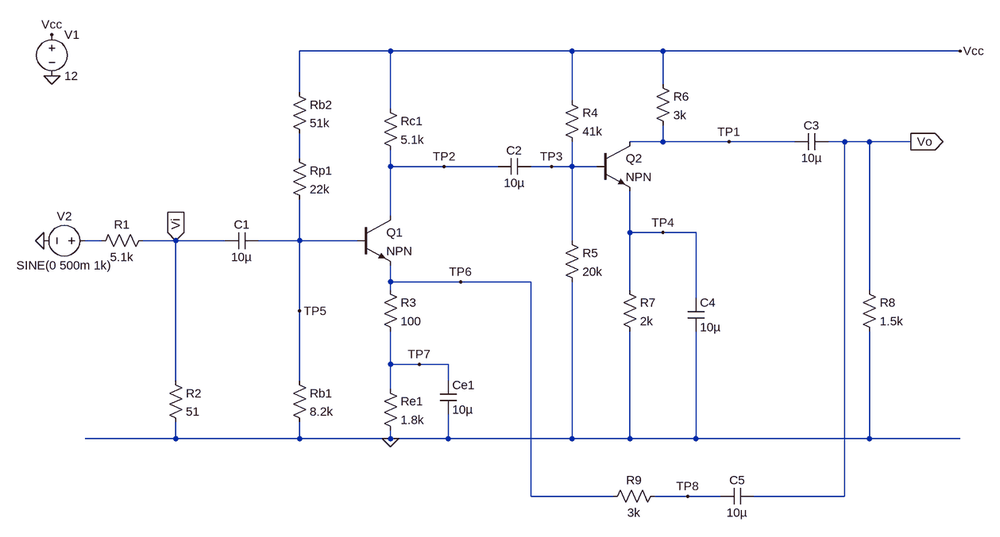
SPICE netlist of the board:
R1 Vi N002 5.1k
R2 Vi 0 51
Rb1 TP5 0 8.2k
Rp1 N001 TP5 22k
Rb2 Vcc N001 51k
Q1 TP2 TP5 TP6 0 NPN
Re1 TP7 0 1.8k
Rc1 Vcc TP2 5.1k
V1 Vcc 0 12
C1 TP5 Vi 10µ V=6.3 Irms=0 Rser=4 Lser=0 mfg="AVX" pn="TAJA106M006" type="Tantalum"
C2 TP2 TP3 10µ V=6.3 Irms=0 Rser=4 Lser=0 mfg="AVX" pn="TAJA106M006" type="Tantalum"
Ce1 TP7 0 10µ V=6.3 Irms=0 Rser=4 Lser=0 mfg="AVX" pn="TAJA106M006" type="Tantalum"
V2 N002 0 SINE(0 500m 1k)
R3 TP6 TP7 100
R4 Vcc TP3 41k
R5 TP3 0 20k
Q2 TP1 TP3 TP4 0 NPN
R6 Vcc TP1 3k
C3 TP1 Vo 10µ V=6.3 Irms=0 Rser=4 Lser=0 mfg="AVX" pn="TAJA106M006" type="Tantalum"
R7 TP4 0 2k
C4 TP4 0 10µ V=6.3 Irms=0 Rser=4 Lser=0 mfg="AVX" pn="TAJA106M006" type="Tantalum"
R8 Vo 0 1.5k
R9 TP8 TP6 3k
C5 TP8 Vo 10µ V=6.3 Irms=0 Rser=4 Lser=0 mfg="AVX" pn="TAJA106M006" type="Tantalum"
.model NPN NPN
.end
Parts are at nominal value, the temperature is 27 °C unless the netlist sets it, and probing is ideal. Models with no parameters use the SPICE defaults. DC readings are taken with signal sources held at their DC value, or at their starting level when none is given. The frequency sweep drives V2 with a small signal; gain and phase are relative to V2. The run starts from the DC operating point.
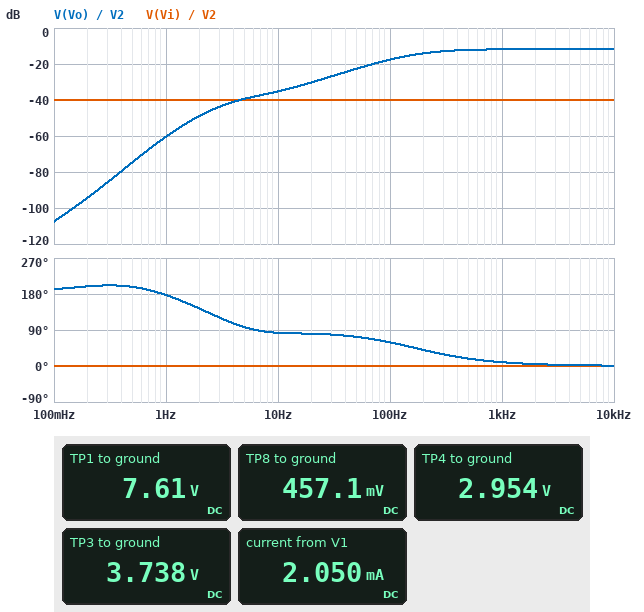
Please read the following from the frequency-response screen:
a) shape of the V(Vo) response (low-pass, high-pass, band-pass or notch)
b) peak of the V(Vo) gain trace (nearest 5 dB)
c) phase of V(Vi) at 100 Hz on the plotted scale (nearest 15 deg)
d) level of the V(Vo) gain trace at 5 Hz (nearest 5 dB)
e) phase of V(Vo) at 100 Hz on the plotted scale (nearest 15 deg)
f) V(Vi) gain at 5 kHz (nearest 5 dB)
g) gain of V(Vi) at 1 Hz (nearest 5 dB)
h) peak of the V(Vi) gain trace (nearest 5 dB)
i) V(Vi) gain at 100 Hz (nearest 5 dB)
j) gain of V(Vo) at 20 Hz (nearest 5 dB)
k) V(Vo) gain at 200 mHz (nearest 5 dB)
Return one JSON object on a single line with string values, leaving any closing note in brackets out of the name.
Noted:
{"shape of the V(Vo) response": "high-pass", "peak of the V(Vo) gain trace": "-10 dB", "phase of V(Vi) at 100 Hz on the plotted scale": "0 deg", "level of the V(Vo) gain trace at 5 Hz": "-40 dB", "phase of V(Vo) at 100 Hz on the plotted scale": "60 deg", "V(Vi) gain at 5 kHz": "-40 dB", "gain of V(Vi) at 1 Hz": "-40 dB", "peak of the V(Vi) gain trace": "-40 dB", "V(Vi) gain at 100 Hz": "-40 dB", "gain of V(Vo) at 20 Hz": "-30 dB", "V(Vo) gain at 200 mHz": "-95 dB"}
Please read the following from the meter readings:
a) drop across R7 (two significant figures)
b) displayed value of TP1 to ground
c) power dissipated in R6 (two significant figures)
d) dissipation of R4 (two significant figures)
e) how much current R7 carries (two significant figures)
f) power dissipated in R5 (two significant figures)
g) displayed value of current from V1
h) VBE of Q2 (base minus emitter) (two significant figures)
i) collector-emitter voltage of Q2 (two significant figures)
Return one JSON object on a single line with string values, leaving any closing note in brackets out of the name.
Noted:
{"drop across R7": "3.0 V", "displayed value of TP1 to ground": "7.61 V", "power dissipated in R6": "6.4 mW", "dissipation of R4": "1.7 mW", "how much current R7 carries": "1.5 mA", "power dissipated in R5": "700 µW", "displayed value of current from V1": "2.050 mA", "VBE of Q2 (base minus emitter)": "780 mV", "collector-emitter voltage of Q2": "4.7 V"}
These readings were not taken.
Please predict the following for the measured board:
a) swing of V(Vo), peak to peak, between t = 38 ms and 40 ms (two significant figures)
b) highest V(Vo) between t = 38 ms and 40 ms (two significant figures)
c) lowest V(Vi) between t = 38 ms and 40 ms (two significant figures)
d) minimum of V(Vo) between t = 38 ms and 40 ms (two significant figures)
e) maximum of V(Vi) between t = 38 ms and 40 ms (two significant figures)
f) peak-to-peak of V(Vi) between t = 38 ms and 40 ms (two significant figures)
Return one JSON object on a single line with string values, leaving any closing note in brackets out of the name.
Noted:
{"swing of V(Vo), peak to peak, between t = 38 ms and 40 ms": "260 mV", "highest V(Vo) between t = 38 ms and 40 ms": "130 mV", "lowest V(Vi) between t = 38 ms and 40 ms": "-4.9 mV", "minimum of V(Vo) between t = 38 ms and 40 ms": "-130 mV", "maximum of V(Vi) between t = 38 ms and 40 ms": "4.9 mV", "peak-to-peak of V(Vi) between t = 38 ms and 40 ms": "9.8 mV"}
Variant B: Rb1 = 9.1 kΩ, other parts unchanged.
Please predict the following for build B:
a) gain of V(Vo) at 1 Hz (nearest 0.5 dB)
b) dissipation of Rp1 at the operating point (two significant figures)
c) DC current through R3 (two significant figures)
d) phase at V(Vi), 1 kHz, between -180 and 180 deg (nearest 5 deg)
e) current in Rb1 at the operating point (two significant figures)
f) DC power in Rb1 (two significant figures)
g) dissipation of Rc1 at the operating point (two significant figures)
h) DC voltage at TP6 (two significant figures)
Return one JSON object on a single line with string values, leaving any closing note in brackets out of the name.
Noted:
{"gain of V(Vo) at 1 Hz": "-59.5 dB", "dissipation of Rp1 at the operating point": "470 µW", "DC current through R3": "300 µA", "phase at V(Vi), 1 kHz, between -180 and 180 deg": "0 deg", "current in Rb1 at the operating point": "140 µA", "DC power in Rb1": "190 µW", "dissipation of Rc1 at the operating point": "440 µW", "DC voltage at TP6": "560 mV"}
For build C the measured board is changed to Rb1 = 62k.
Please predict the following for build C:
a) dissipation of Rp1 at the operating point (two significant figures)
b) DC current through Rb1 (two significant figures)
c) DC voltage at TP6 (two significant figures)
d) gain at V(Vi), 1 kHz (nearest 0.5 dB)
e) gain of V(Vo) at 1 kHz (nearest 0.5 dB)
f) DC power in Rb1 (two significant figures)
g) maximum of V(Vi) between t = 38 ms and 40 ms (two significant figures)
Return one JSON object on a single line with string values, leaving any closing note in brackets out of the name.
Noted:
{"dissipation of Rp1 at the operating point": "260 µW", "DC current through Rb1": "66 µA", "DC voltage at TP6": "3.3 V", "gain at V(Vi), 1 kHz": "-41.0 dB", "gain of V(Vo) at 1 kHz": "-14.0 dB", "DC power in Rb1": "270 µW", "maximum of V(Vi) between t = 38 ms and 40 ms": "4.5 mV"}
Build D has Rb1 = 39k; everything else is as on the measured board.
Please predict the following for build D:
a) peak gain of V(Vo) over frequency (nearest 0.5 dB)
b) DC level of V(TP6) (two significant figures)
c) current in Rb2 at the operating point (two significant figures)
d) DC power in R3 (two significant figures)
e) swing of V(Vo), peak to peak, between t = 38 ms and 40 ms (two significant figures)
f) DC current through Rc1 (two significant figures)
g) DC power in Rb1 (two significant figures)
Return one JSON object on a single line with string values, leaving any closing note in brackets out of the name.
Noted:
{"peak gain of V(Vo) over frequency": "-11.0 dB", "DC level of V(TP6)": "3.0 V", "current in Rb2 at the operating point": "110 µA", "DC power in R3": "250 µW", "swing of V(Vo), peak to peak, between t = 38 ms and 40 ms": "270 mV", "DC current through Rc1": "1.6 mA", "DC power in Rb1": "370 µW"}
